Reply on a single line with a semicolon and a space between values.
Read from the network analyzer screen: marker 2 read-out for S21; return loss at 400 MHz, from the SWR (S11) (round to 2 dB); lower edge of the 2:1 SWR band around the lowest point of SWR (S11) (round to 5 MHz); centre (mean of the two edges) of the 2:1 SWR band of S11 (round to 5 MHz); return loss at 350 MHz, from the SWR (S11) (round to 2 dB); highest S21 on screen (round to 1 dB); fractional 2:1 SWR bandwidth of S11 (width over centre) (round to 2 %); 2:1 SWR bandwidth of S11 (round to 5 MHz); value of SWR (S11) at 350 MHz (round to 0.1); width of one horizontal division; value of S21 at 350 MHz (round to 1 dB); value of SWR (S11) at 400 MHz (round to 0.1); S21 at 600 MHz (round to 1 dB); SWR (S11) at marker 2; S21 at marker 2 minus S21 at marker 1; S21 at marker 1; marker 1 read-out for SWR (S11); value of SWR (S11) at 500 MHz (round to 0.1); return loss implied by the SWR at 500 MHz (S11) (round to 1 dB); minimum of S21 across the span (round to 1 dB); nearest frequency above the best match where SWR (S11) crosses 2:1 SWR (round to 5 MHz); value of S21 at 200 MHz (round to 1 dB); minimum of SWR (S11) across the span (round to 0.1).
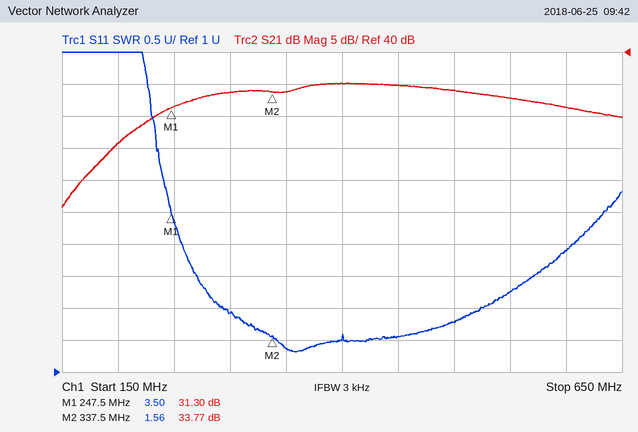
33.77 dB; 14 dB; 295 MHz; 410 MHz; 16 dB; 35 dB; 56 %; 230 MHz; 1.4; 50 MHz; 34 dB; 1.5; 31 dB; 1.56; 2.47 dB; 31.30 dB; 3.50; 1.8; 11 dB; 16 dB; 525 MHz; 26 dB; 1.3
